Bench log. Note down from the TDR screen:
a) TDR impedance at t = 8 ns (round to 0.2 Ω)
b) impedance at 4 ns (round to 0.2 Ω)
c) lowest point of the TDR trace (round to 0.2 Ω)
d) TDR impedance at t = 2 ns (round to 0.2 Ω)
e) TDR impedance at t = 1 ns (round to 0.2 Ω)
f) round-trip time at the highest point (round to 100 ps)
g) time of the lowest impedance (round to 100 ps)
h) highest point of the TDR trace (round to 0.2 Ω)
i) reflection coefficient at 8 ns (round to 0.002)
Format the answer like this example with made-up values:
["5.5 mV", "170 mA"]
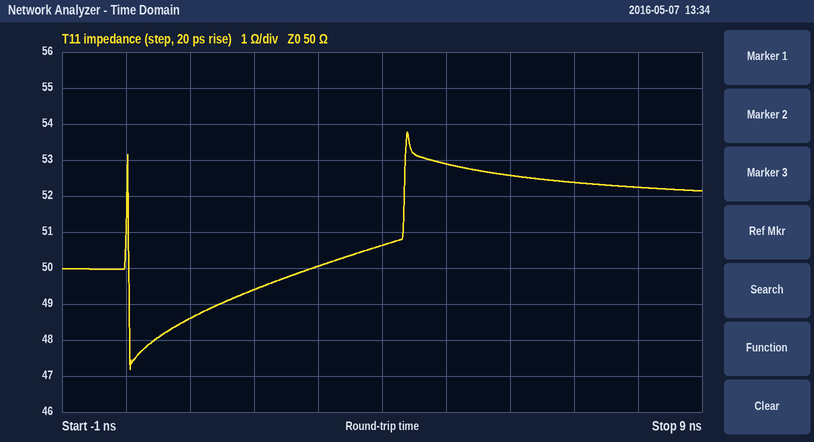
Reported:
["52.2 Ω", "50.6 Ω", "47.2 Ω", "49.4 Ω", "48.6 Ω", "4.4 ns", "100 ps", "53.8 Ω", "+0.022"]
